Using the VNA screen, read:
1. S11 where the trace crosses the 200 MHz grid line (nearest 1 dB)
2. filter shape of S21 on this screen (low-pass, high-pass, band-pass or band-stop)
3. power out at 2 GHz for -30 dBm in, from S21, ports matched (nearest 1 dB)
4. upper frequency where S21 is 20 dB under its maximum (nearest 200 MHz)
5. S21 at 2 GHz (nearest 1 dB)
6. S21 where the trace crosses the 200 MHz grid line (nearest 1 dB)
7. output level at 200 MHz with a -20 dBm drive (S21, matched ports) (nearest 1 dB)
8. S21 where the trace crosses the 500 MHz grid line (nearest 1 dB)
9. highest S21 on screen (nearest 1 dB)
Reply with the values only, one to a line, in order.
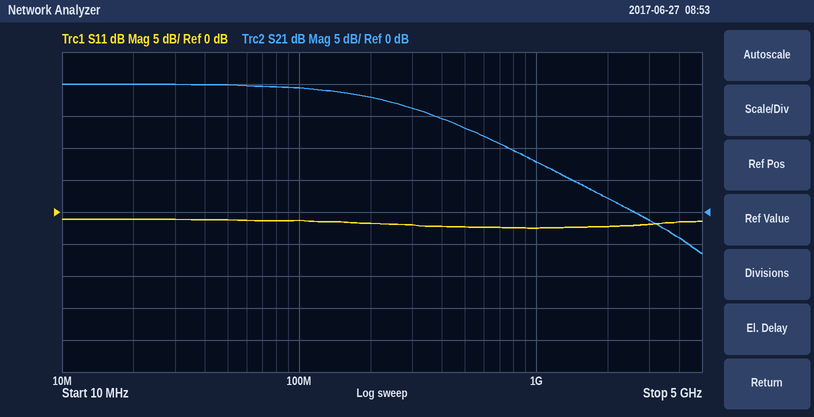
-2 dB
low-pass
-28 dBm
2.6 GHz
2 dB
18 dB
-2 dBm
13 dB
20 dB
